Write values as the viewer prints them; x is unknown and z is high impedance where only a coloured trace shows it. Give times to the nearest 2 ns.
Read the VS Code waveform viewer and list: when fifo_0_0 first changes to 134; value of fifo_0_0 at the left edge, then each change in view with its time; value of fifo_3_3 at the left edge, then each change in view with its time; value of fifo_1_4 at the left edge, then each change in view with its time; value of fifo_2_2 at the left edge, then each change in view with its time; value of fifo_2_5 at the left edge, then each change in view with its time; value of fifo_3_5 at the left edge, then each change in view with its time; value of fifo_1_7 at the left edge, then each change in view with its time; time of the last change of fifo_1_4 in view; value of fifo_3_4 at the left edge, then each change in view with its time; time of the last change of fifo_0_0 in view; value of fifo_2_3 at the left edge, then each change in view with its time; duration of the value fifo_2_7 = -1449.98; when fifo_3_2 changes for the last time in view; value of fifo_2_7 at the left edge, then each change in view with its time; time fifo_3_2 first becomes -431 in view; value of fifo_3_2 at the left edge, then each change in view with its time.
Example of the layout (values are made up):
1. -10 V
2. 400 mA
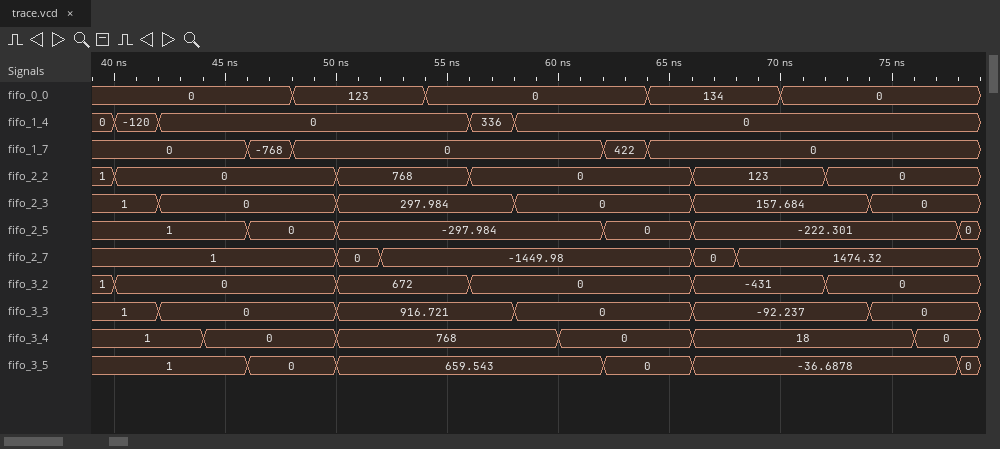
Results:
1. 64 ns
2. 0, 123 at 48 ns, 0 at 54 ns, 134 at 64 ns, 0 at 70 ns
3. 1, 0 at 42 ns, 916.721 at 50 ns, 0 at 58 ns, -92.237 at 66 ns, 0 at 74 ns
4. 0, -120 at 40 ns, 0 at 42 ns, 336 at 56 ns, 0 at 58 ns
5. 1, 0 at 40 ns, 768 at 50 ns, 0 at 56 ns, 123 at 66 ns, 0 at 72 ns
6. 1, 0 at 46 ns, -297.984 at 50 ns, 0 at 62 ns, -222.301 at 66 ns, 0 at 78 ns
7. 1, 0 at 46 ns, 659.543 at 50 ns, 0 at 62 ns, -36.6878 at 66 ns, 0 at 78 ns
8. 0, -768 at 46 ns, 0 at 48 ns, 422 at 62 ns, 0 at 64 ns
9. 58 ns
10. 1, 0 at 44 ns, 768 at 50 ns, 0 at 60 ns, 18 at 66 ns, 0 at 76 ns
11. 70 ns
12. 1, 0 at 42 ns, 297.984 at 50 ns, 0 at 58 ns, 157.684 at 66 ns, 0 at 74 ns
13. 14 ns
14. 72 ns
15. 1, 0 at 50 ns, -1449.98 at 52 ns, 0 at 66 ns, 1474.32 at 68 ns
16. 66 ns
17. 1, 0 at 40 ns, 672 at 50 ns, 0 at 56 ns, -431 at 66 ns, 0 at 72 ns
